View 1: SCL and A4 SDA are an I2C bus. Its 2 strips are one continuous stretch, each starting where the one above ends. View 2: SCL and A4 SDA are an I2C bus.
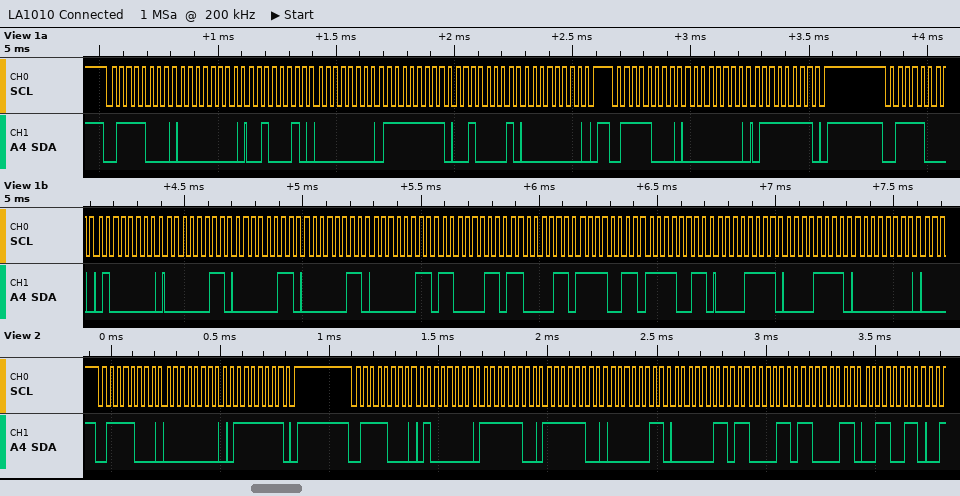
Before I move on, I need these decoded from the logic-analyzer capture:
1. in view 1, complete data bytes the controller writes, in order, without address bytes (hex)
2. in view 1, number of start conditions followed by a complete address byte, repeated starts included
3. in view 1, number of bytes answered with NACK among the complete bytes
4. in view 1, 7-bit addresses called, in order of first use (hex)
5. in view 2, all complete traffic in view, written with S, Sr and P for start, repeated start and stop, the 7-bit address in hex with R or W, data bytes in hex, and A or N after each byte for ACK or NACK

00 22 00 FF 21 00 00 7F 40 03 03 03 03 C3 C3 F3 F3 0F 0F 00
3
0
0x3C
S 3CW A 00 A 7F A P S 3CW A 40 A FC A FC A 03 A 03 A C3 A C3 A 33 A
